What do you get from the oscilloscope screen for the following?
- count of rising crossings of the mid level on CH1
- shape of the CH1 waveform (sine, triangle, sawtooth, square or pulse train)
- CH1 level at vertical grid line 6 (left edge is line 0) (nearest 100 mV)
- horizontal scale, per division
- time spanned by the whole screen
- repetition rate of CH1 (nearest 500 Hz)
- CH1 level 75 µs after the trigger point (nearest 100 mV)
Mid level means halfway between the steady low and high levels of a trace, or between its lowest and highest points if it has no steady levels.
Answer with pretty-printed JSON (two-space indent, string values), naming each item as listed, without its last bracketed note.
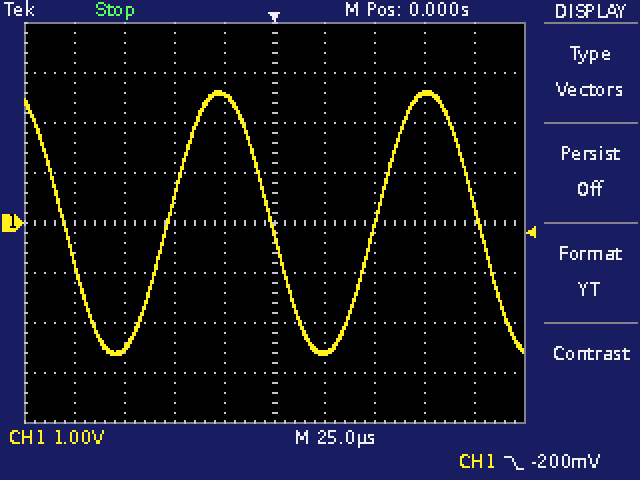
{
  "count of rising crossings of the mid level on CH1": "2",
  "shape of the CH1 waveform": "sine",
  "CH1 level at vertical grid line 6 (left edge is line 0)": "-2.6 V",
  "horizontal scale, per division": "25 µs",
  "time spanned by the whole screen": "250 µs",
  "repetition rate of CH1": "9.5 kHz",
  "CH1 level 75 µs after the trigger point": "2.6 V"
}
